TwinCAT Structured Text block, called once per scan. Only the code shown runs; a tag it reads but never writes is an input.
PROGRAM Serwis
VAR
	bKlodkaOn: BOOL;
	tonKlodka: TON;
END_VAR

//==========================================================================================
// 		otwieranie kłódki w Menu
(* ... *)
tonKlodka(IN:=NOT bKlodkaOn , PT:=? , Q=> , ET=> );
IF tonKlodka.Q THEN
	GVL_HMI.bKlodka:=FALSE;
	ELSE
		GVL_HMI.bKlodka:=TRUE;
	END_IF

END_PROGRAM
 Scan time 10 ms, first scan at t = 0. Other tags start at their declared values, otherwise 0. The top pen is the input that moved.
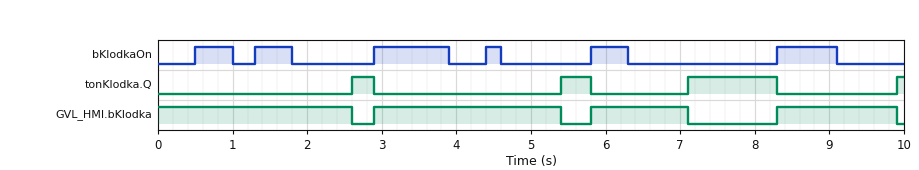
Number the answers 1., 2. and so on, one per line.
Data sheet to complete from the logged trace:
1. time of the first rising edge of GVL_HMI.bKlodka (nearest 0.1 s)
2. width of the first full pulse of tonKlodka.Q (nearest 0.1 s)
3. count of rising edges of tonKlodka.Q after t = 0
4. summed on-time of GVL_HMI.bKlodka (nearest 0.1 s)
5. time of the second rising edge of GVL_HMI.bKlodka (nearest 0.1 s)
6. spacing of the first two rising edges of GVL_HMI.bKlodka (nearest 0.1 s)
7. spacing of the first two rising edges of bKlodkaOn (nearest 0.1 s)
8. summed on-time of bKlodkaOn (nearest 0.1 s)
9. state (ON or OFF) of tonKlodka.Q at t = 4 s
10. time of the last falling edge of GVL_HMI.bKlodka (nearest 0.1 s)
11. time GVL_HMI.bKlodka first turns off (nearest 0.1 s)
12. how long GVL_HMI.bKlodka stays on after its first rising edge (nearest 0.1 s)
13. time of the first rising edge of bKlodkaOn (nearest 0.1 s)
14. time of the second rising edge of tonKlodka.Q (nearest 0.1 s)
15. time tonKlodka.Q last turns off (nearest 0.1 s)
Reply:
1. 2.9 s
2. 0.3 s
3. 4
4. 8.0 s
5. 5.8 s
6. 2.9 s
7. 0.8 s
8. 3.5 s
9. OFF
10. 9.9 s
11. 2.6 s
12. 2.5 s
13. 0.5 s
14. 5.4 s
15. 8.3 s
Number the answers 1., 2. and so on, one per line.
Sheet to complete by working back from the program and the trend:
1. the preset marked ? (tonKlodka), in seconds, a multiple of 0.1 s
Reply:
1. 0.8 s
